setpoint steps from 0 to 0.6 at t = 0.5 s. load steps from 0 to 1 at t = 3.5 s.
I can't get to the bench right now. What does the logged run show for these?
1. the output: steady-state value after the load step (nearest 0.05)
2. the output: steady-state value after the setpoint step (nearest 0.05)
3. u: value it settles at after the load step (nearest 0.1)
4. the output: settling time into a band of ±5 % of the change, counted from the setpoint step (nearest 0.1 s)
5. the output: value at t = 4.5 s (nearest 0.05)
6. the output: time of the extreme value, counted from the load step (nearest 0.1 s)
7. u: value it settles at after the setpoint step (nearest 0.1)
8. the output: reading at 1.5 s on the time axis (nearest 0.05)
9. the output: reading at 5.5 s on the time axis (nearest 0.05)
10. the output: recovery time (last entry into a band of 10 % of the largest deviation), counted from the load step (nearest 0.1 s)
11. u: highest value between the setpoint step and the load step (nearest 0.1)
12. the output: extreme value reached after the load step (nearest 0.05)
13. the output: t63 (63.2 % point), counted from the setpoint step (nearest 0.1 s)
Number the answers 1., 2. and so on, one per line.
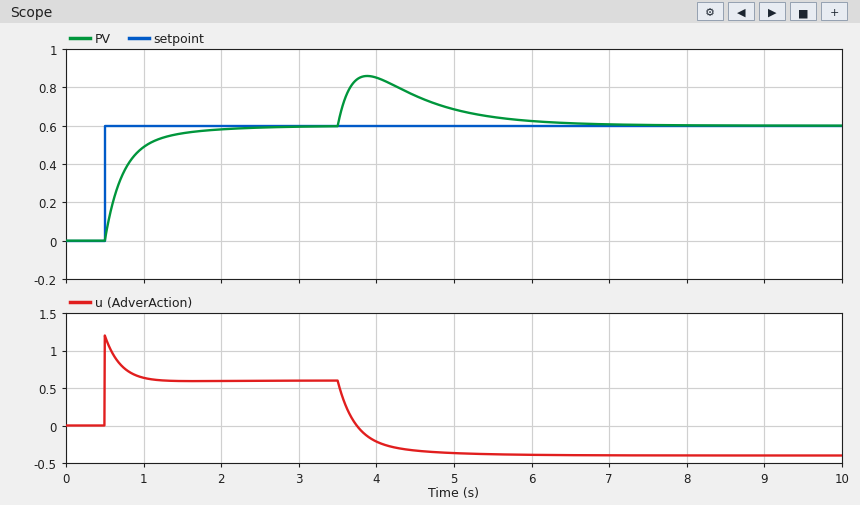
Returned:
1. 0.60
2. 0.60
3. -0.4
4. 1.2 s
5. 0.75
6. 0.4 s
7. 0.6
8. 0.55
9. 0.65
10. 2.4 s
11. 1.2
12. 0.85
13. 0.3 s
